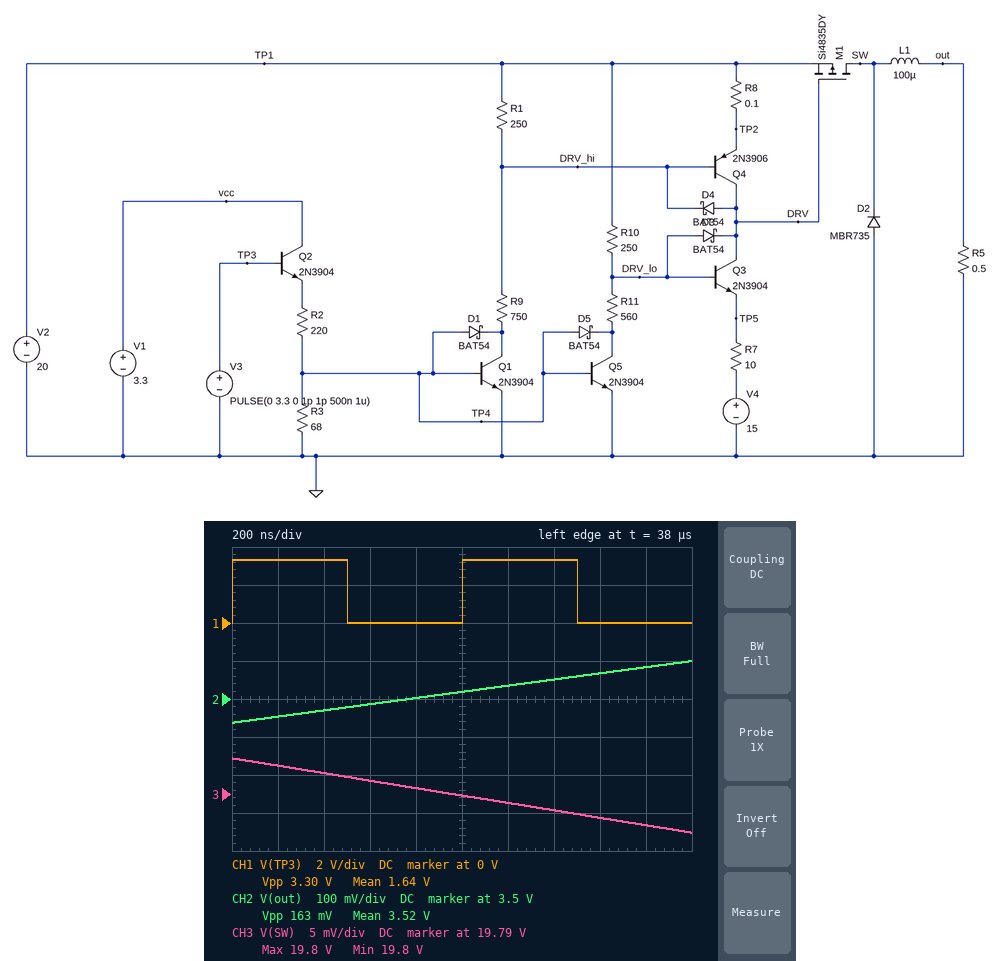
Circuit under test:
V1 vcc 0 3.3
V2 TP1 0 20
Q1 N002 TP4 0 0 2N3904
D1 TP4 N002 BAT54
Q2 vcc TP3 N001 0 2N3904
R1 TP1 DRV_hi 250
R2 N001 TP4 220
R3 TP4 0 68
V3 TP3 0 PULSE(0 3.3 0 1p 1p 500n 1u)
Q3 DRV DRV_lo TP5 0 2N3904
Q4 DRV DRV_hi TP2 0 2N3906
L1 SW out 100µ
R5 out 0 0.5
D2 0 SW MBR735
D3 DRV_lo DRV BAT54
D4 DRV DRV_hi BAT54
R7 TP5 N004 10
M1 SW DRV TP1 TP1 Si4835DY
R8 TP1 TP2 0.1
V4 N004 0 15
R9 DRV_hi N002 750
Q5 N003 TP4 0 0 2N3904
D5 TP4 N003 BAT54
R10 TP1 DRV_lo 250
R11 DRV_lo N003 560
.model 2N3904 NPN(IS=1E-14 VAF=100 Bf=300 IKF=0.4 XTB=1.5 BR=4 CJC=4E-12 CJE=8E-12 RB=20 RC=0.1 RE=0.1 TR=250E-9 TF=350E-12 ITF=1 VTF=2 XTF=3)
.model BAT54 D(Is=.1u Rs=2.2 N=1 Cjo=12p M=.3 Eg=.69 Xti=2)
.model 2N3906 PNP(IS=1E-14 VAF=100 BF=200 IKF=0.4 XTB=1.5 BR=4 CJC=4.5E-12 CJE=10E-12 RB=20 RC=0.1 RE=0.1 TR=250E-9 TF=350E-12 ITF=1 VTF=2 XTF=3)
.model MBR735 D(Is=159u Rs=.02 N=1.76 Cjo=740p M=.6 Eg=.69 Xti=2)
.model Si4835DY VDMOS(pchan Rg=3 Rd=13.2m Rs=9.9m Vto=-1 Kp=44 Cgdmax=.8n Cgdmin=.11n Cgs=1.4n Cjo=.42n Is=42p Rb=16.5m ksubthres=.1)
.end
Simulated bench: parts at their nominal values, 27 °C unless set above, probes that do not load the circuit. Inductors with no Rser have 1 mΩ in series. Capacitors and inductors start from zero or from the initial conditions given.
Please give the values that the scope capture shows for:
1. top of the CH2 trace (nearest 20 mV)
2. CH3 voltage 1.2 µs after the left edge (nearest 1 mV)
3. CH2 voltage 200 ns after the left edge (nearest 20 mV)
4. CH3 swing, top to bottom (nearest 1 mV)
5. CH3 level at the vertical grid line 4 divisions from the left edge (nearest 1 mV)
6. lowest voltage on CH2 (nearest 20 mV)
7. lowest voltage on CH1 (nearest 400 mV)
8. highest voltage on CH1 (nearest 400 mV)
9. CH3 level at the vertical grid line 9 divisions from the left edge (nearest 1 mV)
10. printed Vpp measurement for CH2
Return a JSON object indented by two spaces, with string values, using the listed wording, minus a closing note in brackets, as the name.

{
  "top of the CH2 trace": "3.60 V",
  "CH3 voltage 1.2 µs after the left edge": "19.789 V",
  "CH2 voltage 200 ns after the left edge": "3.46 V",
  "CH3 swing, top to bottom": "10 mV",
  "CH3 level at the vertical grid line 4 divisions from the left edge": "19.791 V",
  "lowest voltage on CH2": "3.44 V",
  "lowest voltage on CH1": "0 V",
  "highest voltage on CH1": "3.2 V",
  "CH3 level at the vertical grid line 9 divisions from the left edge": "19.786 V",
  "printed Vpp measurement for CH2": "163 mV"
}
